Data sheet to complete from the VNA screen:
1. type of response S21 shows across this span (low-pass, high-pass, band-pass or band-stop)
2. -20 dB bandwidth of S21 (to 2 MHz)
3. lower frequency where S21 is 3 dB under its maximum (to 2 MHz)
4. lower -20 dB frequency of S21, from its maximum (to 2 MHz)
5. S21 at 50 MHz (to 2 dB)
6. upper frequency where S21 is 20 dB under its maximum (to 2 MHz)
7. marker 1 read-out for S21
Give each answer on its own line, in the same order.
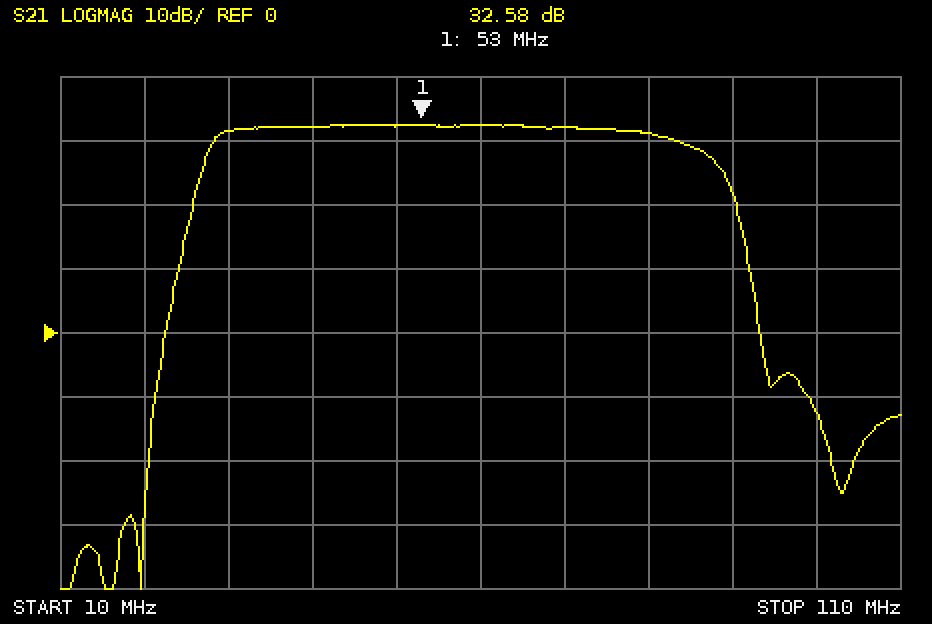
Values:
band-pass
68 MHz
28 MHz
24 MHz
32 dB
92 MHz
32.58 dB
